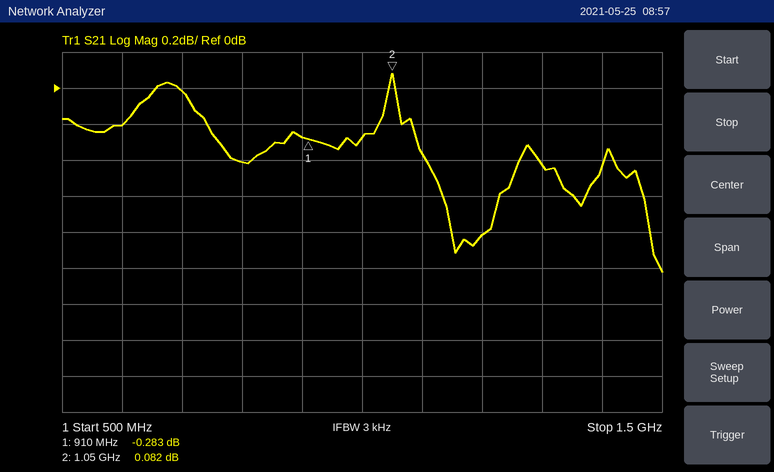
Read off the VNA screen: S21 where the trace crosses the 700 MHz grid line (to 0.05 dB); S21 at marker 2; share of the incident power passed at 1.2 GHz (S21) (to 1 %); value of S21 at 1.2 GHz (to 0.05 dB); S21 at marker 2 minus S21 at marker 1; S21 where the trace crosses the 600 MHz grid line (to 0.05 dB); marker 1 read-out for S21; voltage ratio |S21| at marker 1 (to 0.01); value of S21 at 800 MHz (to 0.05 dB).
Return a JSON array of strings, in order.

["0.00 dB", "0.082 dB", "83 %", "-0.80 dB", "0.365 dB", "-0.20 dB", "-0.283 dB", "0.97", "-0.40 dB"]
